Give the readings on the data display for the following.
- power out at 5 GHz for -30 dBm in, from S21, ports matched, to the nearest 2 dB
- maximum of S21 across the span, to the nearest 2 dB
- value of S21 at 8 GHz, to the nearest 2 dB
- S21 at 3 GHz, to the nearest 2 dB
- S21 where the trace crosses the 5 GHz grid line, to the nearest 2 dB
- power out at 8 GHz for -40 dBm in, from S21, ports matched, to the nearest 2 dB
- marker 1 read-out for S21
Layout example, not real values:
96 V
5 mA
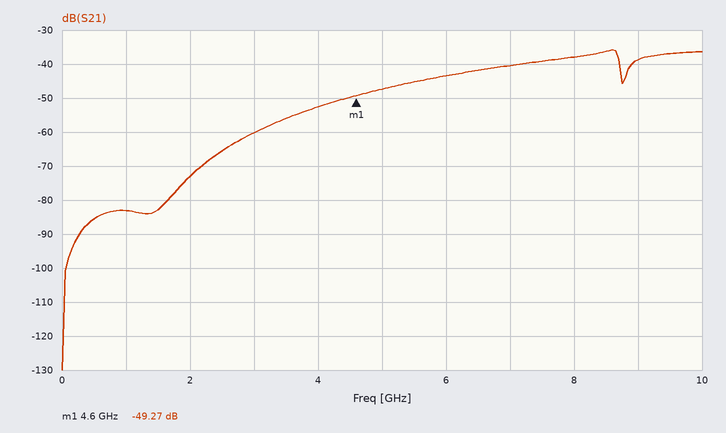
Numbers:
-78 dBm
-36 dB
-38 dB
-60 dB
-48 dB
-78 dBm
-49.27 dB
